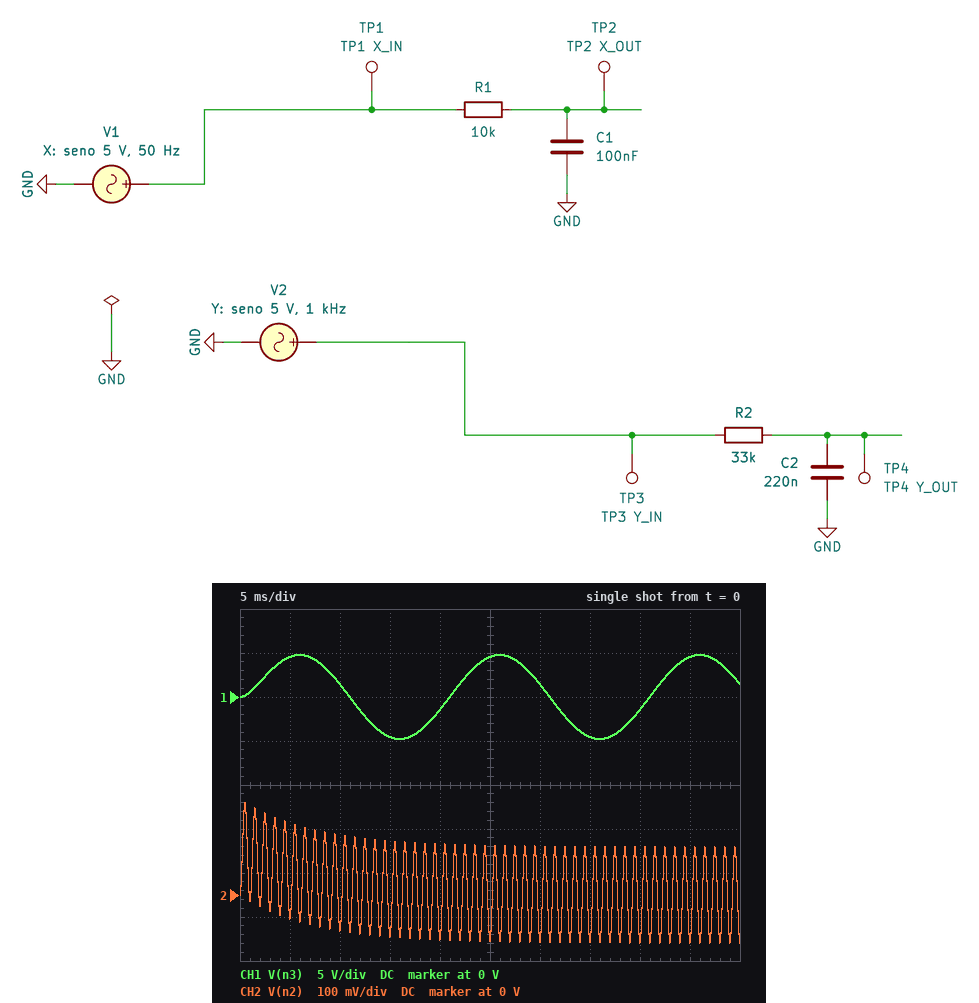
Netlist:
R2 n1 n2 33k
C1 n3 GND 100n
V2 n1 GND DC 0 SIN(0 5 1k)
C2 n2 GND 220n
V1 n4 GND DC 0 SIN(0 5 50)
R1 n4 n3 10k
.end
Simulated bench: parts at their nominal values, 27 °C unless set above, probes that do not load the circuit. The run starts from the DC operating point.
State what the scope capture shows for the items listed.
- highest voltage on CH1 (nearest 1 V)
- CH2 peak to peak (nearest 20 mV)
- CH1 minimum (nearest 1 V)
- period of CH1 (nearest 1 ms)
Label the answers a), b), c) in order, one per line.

a) 5 V
b) 320 mV
c) -5 V
d) 20 ms
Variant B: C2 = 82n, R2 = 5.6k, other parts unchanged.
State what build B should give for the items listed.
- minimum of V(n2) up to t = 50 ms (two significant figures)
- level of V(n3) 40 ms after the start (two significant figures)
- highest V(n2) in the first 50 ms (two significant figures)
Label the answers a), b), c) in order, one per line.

a) -1.6 V
b) -1.4 V
c) 2.2 V
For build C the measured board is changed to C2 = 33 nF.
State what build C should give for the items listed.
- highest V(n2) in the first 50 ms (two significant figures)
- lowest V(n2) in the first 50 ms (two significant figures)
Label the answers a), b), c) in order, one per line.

a) 1.2 V
b) -720 mV
